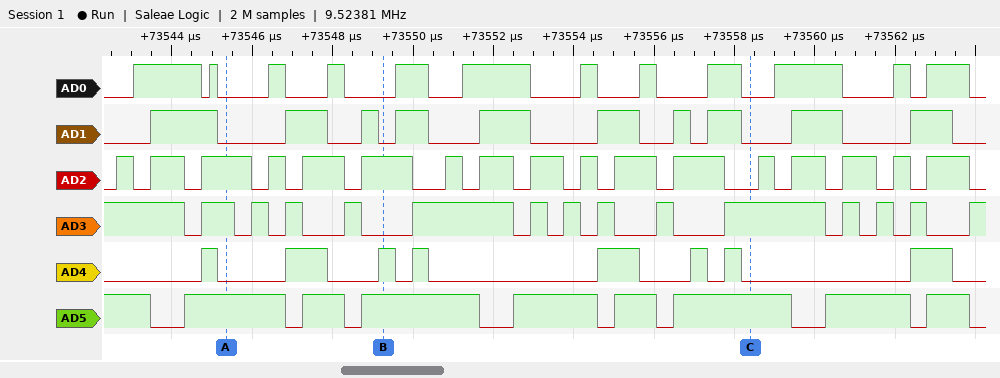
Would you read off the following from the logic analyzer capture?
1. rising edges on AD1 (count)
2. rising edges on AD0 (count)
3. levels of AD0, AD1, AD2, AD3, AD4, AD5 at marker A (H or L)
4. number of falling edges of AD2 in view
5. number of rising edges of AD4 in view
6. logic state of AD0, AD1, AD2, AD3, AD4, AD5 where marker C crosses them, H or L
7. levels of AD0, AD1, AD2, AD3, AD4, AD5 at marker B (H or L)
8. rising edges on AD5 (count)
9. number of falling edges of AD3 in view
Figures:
10
12
AD0=L, AD1=L, AD2=H, AD3=H, AD4=L, AD5=H
17
8
AD0=L, AD1=L, AD2=L, AD3=H, AD4=L, AD5=H
AD0=L, AD1=L, AD2=H, AD3=L, AD4=H, AD5=H
8
14
